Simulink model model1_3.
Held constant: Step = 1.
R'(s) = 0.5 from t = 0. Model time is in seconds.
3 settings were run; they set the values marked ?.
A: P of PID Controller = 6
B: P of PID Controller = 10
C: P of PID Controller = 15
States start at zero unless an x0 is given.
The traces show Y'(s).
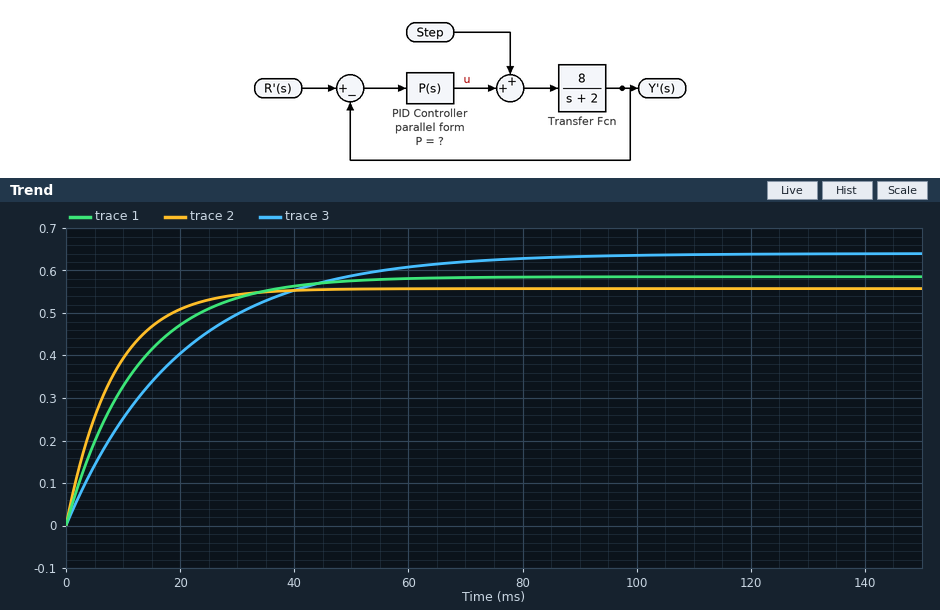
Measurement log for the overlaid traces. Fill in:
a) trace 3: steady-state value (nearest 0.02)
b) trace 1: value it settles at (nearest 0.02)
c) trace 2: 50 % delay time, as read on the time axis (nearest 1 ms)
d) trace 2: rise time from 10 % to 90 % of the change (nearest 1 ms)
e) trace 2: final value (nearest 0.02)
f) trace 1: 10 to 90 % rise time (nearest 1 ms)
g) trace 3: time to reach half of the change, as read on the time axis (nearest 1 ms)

0.64
0.58
6 ms
18 ms
0.56
27 ms
14 ms
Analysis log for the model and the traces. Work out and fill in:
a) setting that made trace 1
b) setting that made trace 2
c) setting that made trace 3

B
C
A
